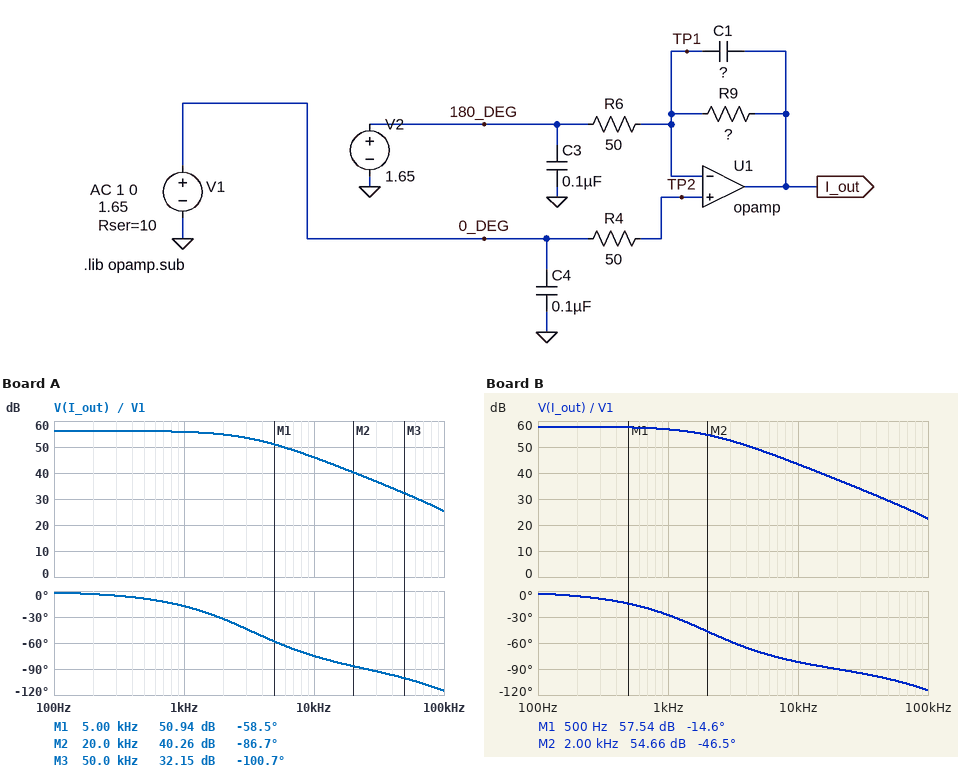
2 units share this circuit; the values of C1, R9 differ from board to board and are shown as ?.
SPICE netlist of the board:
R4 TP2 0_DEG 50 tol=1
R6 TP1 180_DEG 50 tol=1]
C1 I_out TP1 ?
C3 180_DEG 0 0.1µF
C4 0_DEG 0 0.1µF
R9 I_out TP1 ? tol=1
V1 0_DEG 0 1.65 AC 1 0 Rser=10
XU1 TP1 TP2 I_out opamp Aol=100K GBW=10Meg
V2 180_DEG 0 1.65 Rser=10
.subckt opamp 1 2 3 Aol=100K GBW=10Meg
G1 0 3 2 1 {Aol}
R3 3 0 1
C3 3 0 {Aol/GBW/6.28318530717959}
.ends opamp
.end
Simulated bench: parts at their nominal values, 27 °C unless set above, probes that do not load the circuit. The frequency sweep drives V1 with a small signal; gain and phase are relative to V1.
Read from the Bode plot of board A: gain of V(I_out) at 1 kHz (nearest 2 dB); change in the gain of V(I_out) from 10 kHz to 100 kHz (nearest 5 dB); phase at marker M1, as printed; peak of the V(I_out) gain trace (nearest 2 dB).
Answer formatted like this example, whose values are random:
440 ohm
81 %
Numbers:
56 dB
-20 dB
-58.5 deg
56 dB
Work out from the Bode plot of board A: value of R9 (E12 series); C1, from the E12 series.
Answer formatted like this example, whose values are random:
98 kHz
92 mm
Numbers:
39 kΩ
1 nF
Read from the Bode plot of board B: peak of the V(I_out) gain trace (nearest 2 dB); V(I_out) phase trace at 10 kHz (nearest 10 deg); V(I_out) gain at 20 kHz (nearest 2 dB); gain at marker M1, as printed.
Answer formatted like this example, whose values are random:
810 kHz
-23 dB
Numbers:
58 dB
-80 deg
38 dB
57.54 dB
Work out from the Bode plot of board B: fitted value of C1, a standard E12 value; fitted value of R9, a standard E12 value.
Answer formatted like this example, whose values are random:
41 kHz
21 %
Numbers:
1.5 nF
47 kΩ
